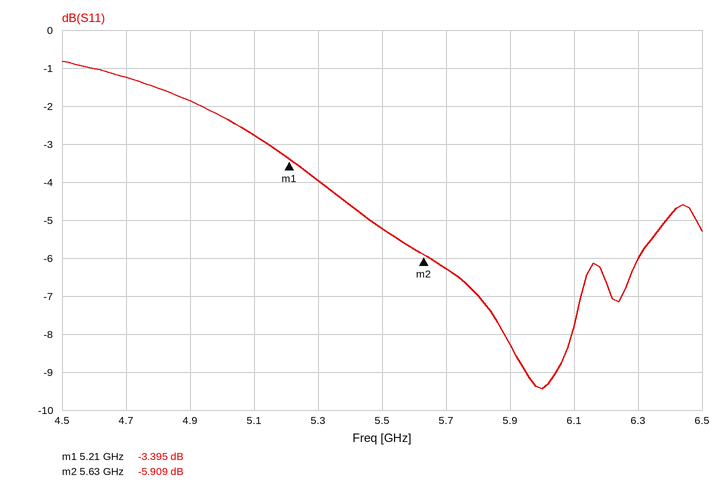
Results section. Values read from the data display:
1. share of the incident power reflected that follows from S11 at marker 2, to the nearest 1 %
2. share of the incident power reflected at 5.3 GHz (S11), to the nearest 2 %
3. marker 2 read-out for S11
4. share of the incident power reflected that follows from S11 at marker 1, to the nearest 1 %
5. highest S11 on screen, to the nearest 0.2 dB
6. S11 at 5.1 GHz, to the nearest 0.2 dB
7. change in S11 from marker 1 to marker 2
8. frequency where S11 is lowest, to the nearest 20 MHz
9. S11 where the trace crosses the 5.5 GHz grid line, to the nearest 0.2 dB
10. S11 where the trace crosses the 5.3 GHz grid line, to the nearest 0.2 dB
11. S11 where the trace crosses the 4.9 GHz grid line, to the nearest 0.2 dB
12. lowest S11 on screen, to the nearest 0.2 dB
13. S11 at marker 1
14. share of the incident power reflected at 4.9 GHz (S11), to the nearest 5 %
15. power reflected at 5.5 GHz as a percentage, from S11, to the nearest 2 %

26 %
40 %
-5.909 dB
46 %
-0.8 dB
-2.8 dB
-2.514 dB
6.00 GHz
-5.2 dB
-4.0 dB
-1.8 dB
-9.4 dB
-3.395 dB
65 %
30 %
